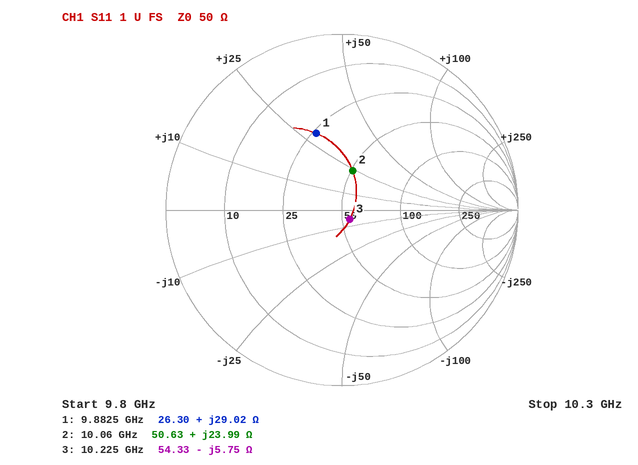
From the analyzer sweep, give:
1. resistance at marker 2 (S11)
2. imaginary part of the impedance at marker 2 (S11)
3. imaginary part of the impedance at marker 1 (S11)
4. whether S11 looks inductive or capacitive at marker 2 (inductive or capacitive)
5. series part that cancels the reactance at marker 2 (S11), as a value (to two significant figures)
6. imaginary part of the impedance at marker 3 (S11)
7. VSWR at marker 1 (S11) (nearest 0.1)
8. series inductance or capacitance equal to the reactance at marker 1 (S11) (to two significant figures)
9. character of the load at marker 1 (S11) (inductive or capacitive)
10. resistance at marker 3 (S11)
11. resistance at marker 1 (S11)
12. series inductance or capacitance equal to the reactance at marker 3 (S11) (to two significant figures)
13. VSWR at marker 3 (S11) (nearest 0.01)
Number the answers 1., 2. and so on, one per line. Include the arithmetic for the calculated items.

1. 50.63 Ω
2. +23.99 Ω
3. +29.02 Ω
4. inductive
5. C = 1/(2π × 10.06 GHz × 23.99 Ω) ≈ 659 fF, so 660 fF to two significant figures
6. -5.75 Ω
7. 2.7
8. L = 29.02 Ω/(2π × 9.8825 GHz) ≈ 467 pH, so 470 pH to two significant figures
9. inductive
10. 54.33 Ω
11. 26.30 Ω
12. C = 1/(2π × 10.225 GHz × 5.75 Ω) ≈ 2.7 pF
13. 1.15
